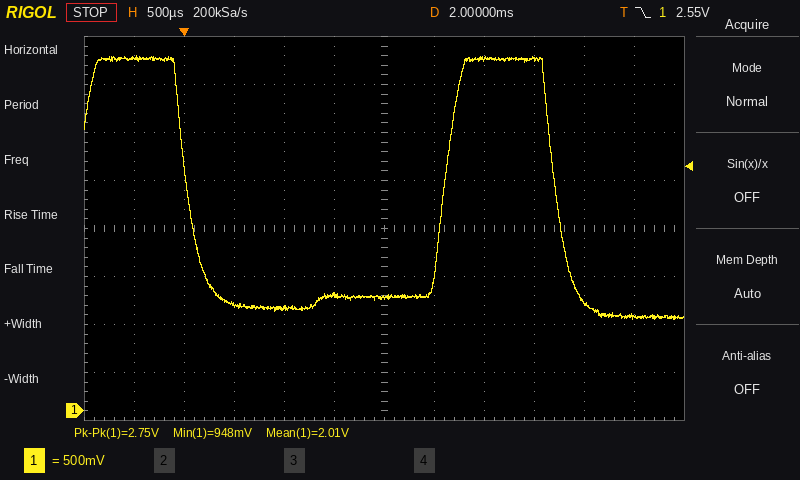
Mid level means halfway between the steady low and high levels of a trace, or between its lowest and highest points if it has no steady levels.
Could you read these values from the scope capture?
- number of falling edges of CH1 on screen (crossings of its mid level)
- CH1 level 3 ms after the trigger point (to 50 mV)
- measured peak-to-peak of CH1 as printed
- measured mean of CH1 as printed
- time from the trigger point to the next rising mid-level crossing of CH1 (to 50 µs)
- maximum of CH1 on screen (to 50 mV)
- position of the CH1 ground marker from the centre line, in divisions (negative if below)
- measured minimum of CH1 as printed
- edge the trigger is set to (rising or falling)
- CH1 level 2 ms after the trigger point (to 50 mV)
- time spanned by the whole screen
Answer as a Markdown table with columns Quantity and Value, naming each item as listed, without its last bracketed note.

| Quantity | Value |
|---|---|
| number of falling edges of CH1 on screen | 2 |
| CH1 level 3 ms after the trigger point | 3.65 V |
| measured peak-to-peak of CH1 as printed | 2.75 V |
| measured mean of CH1 as printed | 2.01 V |
| time from the trigger point to the next rising mid-level crossing of CH1 | 2.60 ms |
| maximum of CH1 on screen | 3.70 V |
| position of the CH1 ground marker from the centre line, in divisions | -3.8 div |
| measured minimum of CH1 as printed | 948 mV |
| edge the trigger is set to | falling |
| CH1 level 2 ms after the trigger point | 1.20 V |
| time spanned by the whole screen | 6 ms |
